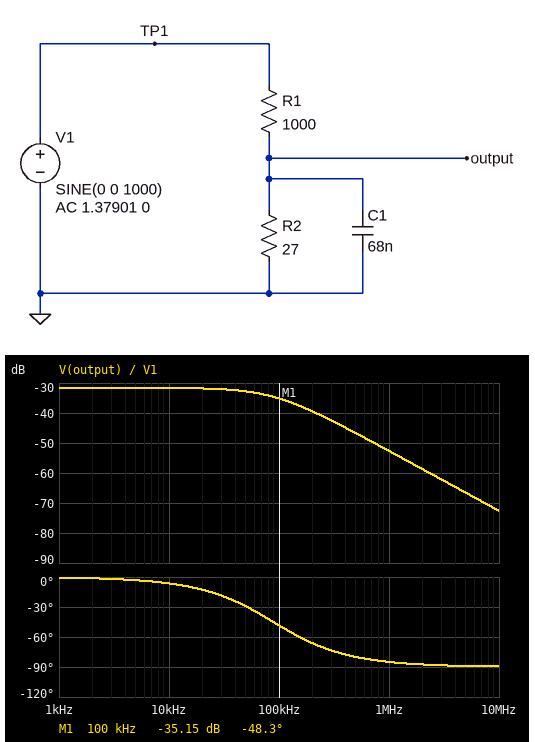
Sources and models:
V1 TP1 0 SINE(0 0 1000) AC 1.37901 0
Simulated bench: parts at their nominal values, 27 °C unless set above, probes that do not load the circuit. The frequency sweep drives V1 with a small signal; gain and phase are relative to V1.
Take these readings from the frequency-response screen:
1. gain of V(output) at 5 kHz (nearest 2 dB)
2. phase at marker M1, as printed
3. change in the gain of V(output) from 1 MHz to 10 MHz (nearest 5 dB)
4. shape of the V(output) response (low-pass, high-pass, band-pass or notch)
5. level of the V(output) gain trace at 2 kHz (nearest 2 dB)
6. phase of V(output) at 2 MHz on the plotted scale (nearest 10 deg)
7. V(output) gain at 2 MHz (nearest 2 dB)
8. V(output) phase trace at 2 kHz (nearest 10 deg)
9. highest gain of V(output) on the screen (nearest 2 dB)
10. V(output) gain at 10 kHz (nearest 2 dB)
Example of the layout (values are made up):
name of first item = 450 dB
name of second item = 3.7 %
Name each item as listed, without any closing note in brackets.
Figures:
gain of V(output) at 5 kHz = -32 dB
phase at marker M1, as printed = -48.3 deg
change in the gain of V(output) from 1 MHz to 10 MHz = -20 dB
shape of the V(output) response = low-pass
level of the V(output) gain trace at 2 kHz = -32 dB
phase of V(output) at 2 MHz on the plotted scale = -90 deg
V(output) gain at 2 MHz = -58 dB
V(output) phase trace at 2 kHz = 0 deg
highest gain of V(output) on the screen = -32 dB
V(output) gain at 10 kHz = -32 dB
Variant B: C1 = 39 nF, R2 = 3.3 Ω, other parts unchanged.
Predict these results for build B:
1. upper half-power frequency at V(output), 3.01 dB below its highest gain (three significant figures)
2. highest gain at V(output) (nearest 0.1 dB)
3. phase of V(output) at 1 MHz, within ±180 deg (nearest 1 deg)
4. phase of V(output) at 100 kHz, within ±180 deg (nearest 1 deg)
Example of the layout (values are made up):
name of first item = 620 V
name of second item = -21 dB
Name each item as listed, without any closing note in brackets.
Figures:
upper half-power frequency at V(output), 3.01 dB below its highest gain = 1.24 MHz
highest gain at V(output) = -49.7 dB
phase of V(output) at 1 MHz, within ±180 deg = -39 deg
phase of V(output) at 100 kHz, within ±180 deg = -5 deg
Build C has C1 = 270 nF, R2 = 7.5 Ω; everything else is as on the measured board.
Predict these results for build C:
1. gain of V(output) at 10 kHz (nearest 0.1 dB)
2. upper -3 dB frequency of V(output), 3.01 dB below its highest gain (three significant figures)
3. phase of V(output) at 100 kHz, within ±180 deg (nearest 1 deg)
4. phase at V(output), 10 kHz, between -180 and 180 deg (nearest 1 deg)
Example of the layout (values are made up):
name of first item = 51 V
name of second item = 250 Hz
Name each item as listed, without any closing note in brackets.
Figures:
gain of V(output) at 10 kHz = -42.6 dB
upper -3 dB frequency of V(output), 3.01 dB below its highest gain = 79.2 kHz
phase of V(output) at 100 kHz, within ±180 deg = -52 deg
phase at V(output), 10 kHz, between -180 and 180 deg = -7 deg
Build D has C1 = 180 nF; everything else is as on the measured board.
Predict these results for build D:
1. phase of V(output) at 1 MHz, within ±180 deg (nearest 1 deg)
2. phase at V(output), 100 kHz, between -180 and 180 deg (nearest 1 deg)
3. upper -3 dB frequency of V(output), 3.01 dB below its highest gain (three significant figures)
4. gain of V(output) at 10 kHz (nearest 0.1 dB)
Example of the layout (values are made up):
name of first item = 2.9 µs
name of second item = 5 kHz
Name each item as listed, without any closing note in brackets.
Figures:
phase of V(output) at 1 MHz, within ±180 deg = -88 deg
phase at V(output), 100 kHz, between -180 and 180 deg = -71 deg
upper -3 dB frequency of V(output), 3.01 dB below its highest gain = 33.6 kHz
gain of V(output) at 10 kHz = -32.0 dB
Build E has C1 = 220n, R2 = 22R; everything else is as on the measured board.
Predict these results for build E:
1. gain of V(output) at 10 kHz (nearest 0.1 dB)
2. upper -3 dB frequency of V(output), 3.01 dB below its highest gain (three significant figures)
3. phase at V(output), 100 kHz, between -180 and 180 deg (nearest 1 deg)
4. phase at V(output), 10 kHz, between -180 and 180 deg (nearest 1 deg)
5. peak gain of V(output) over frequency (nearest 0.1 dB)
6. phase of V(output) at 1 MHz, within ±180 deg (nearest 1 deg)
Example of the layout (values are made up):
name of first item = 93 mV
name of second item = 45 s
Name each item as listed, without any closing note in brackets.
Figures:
gain of V(output) at 10 kHz = -33.7 dB
upper -3 dB frequency of V(output), 3.01 dB below its highest gain = 33.6 kHz
phase at V(output), 100 kHz, between -180 and 180 deg = -71 deg
phase at V(output), 10 kHz, between -180 and 180 deg = -17 deg
peak gain of V(output) over frequency = -33.3 dB
phase of V(output) at 1 MHz, within ±180 deg = -88 deg
